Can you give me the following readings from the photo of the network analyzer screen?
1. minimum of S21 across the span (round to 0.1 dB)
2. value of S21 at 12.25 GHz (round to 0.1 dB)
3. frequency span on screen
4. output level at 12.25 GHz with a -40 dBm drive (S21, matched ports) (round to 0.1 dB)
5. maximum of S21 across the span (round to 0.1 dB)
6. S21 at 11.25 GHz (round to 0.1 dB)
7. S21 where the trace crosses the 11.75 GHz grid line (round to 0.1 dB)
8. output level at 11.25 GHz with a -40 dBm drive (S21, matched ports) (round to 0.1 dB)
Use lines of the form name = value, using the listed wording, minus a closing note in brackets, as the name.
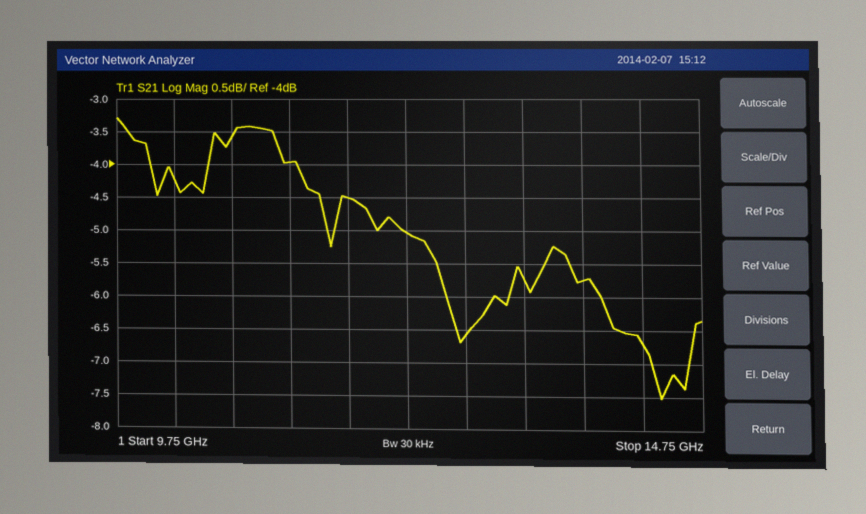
minimum of S21 across the span = -7.5 dB
value of S21 at 12.25 GHz = -5.0 dB
frequency span on screen = 5 GHz
output level at 12.25 GHz with a -40 dBm drive (S21, matched ports) = -45.0 dBm
maximum of S21 across the span = -3.3 dB
S21 at 11.25 GHz = -4.0 dB
S21 where the trace crosses the 11.75 GHz grid line = -4.5 dB
output level at 11.25 GHz with a -40 dBm drive (S21, matched ports) = -44.0 dBm
